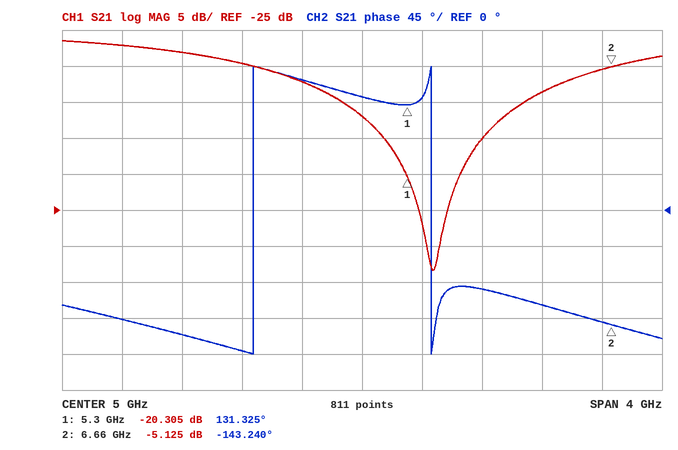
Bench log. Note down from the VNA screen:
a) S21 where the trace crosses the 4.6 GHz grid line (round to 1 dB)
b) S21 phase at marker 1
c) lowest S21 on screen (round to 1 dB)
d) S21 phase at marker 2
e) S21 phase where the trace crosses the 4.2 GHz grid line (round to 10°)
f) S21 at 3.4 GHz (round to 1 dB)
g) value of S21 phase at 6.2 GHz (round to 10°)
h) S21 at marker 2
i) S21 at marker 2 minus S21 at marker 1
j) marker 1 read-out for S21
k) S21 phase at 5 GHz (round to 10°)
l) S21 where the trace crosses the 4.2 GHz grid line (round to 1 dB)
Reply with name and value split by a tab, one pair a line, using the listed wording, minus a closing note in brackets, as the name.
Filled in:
S21 where the trace crosses the 4.6 GHz grid line	-7 dB
S21 phase at marker 1	131.325°
lowest S21 on screen	-33 dB
S21 phase at marker 2	-143.240°
S21 phase where the trace crosses the 4.2 GHz grid line	-180°
S21 at 3.4 GHz	-2 dB
value of S21 phase at 6.2 GHz	-120°
S21 at marker 2	-5.125 dB
S21 at marker 2 minus S21 at marker 1	15.180 dB
marker 1 read-out for S21	-20.305 dB
S21 phase at 5 GHz	140°
S21 where the trace crosses the 4.2 GHz grid line	-5 dB
